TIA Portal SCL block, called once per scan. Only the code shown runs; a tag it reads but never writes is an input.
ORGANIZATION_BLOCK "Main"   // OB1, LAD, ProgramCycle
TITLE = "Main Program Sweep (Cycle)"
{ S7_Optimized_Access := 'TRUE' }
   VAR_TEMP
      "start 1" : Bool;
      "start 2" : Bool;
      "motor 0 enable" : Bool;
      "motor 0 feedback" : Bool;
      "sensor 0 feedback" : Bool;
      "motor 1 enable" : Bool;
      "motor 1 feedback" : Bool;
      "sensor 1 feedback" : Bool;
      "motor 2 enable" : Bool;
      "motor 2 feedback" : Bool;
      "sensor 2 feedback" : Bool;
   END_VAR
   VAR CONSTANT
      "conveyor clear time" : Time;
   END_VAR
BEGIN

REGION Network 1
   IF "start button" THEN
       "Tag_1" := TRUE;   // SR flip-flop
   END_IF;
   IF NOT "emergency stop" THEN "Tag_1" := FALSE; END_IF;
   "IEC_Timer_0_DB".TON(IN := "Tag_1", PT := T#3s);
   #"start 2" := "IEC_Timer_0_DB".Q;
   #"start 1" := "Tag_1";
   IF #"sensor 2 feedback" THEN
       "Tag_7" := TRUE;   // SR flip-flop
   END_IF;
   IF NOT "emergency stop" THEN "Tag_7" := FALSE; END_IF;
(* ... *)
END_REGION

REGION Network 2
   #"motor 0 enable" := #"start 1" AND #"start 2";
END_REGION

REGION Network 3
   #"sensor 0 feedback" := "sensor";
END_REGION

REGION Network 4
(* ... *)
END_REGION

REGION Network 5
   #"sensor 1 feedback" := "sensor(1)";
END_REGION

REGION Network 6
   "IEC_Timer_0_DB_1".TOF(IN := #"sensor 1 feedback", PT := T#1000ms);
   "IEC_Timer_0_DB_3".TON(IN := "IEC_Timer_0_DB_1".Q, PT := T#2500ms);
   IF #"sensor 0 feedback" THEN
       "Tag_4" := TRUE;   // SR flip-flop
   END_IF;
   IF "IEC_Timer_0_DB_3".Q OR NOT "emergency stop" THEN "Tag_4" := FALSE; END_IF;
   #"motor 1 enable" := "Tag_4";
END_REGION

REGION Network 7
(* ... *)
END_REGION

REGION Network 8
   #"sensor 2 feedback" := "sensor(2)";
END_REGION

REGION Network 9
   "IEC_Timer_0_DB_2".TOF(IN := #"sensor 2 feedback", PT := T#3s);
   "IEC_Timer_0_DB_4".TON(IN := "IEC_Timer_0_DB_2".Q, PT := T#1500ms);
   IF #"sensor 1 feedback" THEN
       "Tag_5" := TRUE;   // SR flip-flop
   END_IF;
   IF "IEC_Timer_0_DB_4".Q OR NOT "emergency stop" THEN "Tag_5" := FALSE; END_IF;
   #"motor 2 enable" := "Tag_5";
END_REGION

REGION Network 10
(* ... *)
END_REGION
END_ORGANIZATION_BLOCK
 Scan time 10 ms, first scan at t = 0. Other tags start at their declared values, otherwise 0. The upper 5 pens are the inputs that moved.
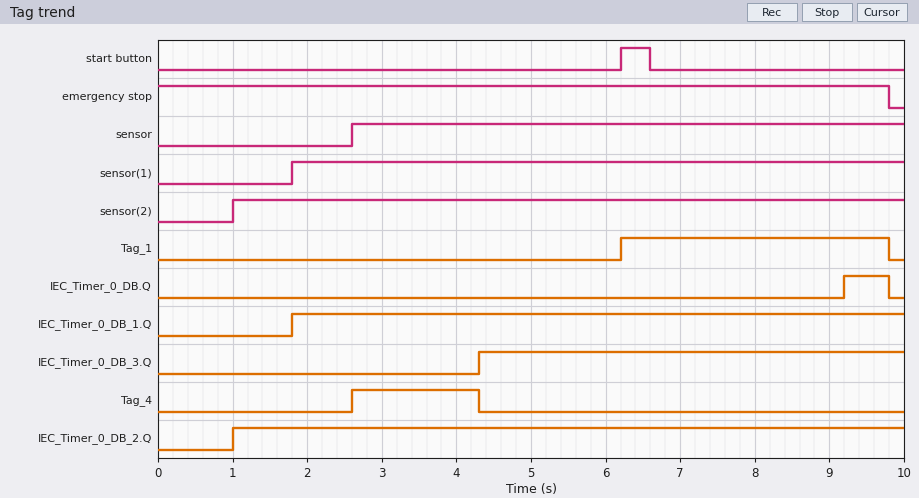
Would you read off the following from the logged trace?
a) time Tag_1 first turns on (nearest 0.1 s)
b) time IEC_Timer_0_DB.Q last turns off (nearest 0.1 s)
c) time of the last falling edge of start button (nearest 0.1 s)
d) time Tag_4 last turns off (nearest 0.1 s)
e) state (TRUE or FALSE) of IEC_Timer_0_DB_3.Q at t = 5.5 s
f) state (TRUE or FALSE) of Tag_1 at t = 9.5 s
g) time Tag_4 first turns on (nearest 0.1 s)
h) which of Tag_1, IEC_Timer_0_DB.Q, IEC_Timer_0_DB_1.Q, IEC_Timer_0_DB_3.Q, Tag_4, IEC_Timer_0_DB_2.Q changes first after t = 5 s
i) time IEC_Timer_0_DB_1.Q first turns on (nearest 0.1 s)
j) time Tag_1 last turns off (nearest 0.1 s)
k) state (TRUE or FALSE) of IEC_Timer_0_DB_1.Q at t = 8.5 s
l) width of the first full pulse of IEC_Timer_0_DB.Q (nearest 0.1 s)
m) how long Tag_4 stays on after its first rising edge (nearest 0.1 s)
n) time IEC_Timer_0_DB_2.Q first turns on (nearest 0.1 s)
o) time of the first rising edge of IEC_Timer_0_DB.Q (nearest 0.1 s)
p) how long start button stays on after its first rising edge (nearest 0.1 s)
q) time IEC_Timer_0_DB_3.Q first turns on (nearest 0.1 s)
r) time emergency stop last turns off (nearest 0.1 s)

6.2 s
9.8 s
6.6 s
4.3 s
TRUE
TRUE
2.6 s
Tag_1
1.8 s
9.8 s
TRUE
0.6 s
1.7 s
1.0 s
9.2 s
0.4 s
4.3 s
9.8 s
